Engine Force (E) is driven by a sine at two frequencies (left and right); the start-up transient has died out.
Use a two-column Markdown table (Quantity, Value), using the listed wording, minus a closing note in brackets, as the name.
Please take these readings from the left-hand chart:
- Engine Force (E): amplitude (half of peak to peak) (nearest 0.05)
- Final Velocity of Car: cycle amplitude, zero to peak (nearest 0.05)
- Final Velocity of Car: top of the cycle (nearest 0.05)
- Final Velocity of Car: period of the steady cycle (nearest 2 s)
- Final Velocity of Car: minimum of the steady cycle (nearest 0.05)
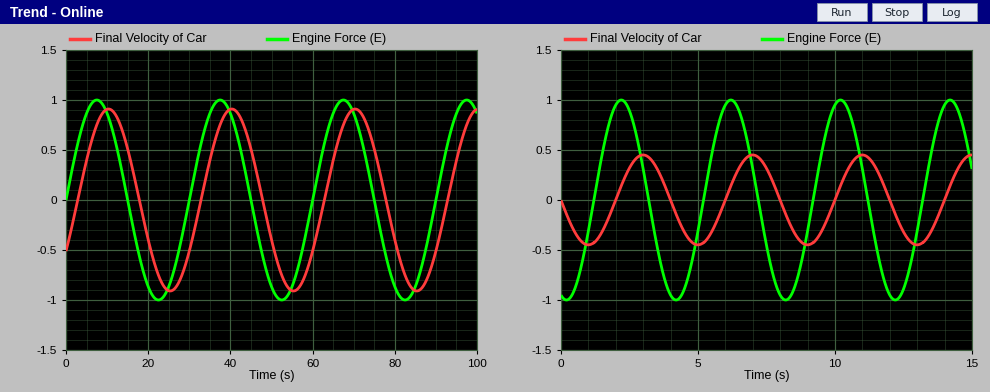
| Quantity | Value |
|---|---|
| Engine Force (E): amplitude (half of peak to peak) | 1.00 |
| Final Velocity of Car: cycle amplitude, zero to peak | 0.90 |
| Final Velocity of Car: top of the cycle | 0.90 |
| Final Velocity of Car: period of the steady cycle | 30 s |
| Final Velocity of Car: minimum of the steady cycle | -0.90 |
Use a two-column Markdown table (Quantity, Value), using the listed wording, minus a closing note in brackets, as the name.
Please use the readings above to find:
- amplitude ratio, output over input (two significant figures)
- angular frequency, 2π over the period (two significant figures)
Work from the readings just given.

| Quantity | Value |
|---|---|
| amplitude ratio, output over input | 0.90 |
| angular frequency, 2π over the period | 0.21 rad/s |
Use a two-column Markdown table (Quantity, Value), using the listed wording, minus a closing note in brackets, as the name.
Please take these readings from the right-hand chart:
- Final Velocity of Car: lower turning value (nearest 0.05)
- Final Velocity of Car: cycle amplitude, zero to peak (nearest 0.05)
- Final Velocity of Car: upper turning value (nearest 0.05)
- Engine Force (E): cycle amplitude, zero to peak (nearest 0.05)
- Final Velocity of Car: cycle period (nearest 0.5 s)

| Quantity | Value |
|---|---|
| Final Velocity of Car: lower turning value | -0.45 |
| Final Velocity of Car: cycle amplitude, zero to peak | 0.45 |
| Final Velocity of Car: upper turning value | 0.45 |
| Engine Force (E): cycle amplitude, zero to peak | 1.00 |
| Final Velocity of Car: cycle period | 4.0 s |
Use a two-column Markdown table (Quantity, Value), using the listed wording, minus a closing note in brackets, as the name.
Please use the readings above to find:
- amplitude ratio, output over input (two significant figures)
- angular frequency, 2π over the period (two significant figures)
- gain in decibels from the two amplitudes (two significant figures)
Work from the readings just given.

| Quantity | Value |
|---|---|
| amplitude ratio, output over input | 0.45 |
| angular frequency, 2π over the period | 1.6 rad/s |
| gain in decibels from the two amplitudes | -6.9 dB |
